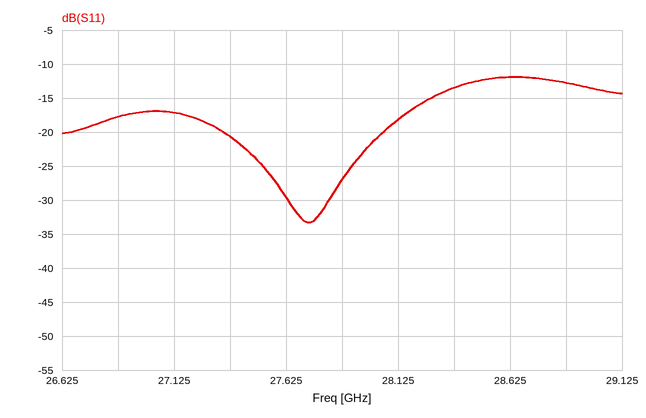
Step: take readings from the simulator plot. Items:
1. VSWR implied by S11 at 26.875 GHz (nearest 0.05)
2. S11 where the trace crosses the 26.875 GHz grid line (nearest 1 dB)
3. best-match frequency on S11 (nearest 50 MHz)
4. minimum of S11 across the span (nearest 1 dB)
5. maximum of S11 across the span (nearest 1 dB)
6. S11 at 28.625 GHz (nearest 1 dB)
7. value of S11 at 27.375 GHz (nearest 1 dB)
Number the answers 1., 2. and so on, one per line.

1. 1.30
2. -18 dB
3. 27.70 GHz
4. -33 dB
5. -12 dB
6. -12 dB
7. -21 dB
